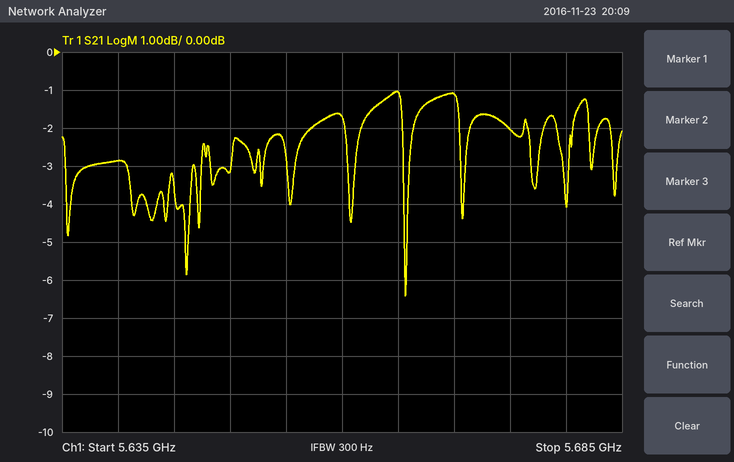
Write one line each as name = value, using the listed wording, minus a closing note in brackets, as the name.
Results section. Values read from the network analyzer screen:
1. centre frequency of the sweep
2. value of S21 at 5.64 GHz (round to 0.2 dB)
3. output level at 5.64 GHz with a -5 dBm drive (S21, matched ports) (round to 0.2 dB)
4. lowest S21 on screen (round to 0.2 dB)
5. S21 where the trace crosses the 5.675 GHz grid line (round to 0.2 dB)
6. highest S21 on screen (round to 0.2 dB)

centre frequency of the sweep = 5.66 GHz
value of S21 at 5.64 GHz = -2.8 dB
output level at 5.64 GHz with a -5 dBm drive (S21, matched ports) = -7.8 dBm
lowest S21 on screen = -6.4 dB
S21 where the trace crosses the 5.675 GHz grid line = -2.0 dB
highest S21 on screen = -1.0 dB
